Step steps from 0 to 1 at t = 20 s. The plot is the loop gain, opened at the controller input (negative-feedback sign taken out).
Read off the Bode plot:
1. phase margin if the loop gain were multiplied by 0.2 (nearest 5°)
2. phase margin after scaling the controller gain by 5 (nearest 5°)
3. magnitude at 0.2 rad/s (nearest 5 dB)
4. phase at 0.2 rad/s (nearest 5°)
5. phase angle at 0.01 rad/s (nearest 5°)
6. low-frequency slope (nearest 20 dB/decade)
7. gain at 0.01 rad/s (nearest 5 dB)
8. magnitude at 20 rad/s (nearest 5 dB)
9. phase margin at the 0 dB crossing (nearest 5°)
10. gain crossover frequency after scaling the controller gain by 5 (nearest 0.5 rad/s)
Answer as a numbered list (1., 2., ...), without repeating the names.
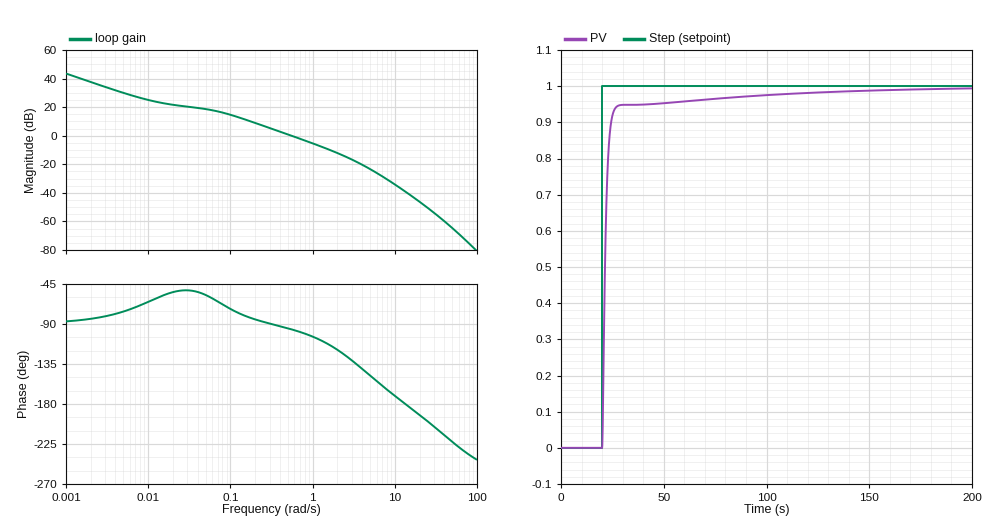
1. 105°
2. 55°
3. 10 dB
4. -85°
5. -65°
6. -20 dB/decade
7. 25 dB
8. -45 dB
9. 85°
10. 2.5 rad/s
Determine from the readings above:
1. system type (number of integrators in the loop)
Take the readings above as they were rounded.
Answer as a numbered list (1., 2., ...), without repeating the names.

1. 1
